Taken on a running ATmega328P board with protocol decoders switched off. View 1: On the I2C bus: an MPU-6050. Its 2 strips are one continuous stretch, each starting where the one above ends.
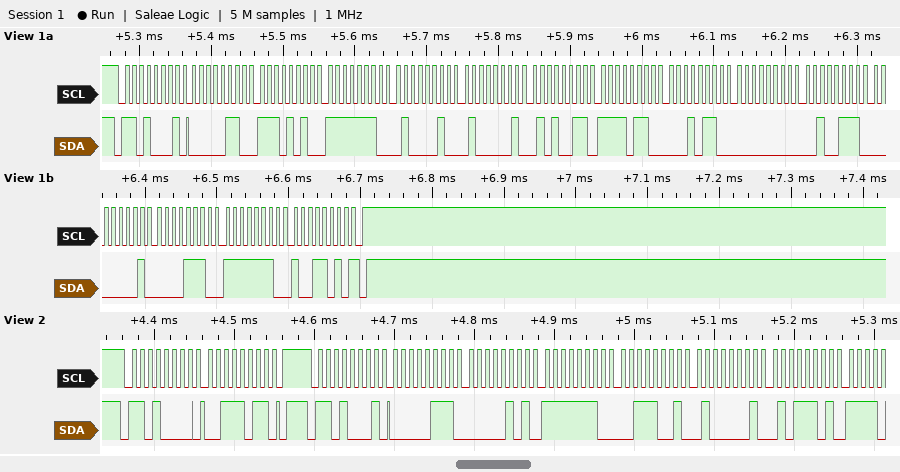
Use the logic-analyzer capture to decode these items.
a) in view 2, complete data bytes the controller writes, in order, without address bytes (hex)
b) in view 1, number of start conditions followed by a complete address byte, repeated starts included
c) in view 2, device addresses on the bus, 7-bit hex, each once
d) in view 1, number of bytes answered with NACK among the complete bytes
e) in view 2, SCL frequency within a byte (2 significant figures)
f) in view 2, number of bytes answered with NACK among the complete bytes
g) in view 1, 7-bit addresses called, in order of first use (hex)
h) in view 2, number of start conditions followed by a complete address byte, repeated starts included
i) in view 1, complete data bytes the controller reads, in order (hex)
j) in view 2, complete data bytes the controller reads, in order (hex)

3B
1
0x68
1
100 kHz
0
0x68
2
06 EA FE 42 41 53 F6 16 00 27 01 0E FE 9A
07 05 FE 39 41 5D
